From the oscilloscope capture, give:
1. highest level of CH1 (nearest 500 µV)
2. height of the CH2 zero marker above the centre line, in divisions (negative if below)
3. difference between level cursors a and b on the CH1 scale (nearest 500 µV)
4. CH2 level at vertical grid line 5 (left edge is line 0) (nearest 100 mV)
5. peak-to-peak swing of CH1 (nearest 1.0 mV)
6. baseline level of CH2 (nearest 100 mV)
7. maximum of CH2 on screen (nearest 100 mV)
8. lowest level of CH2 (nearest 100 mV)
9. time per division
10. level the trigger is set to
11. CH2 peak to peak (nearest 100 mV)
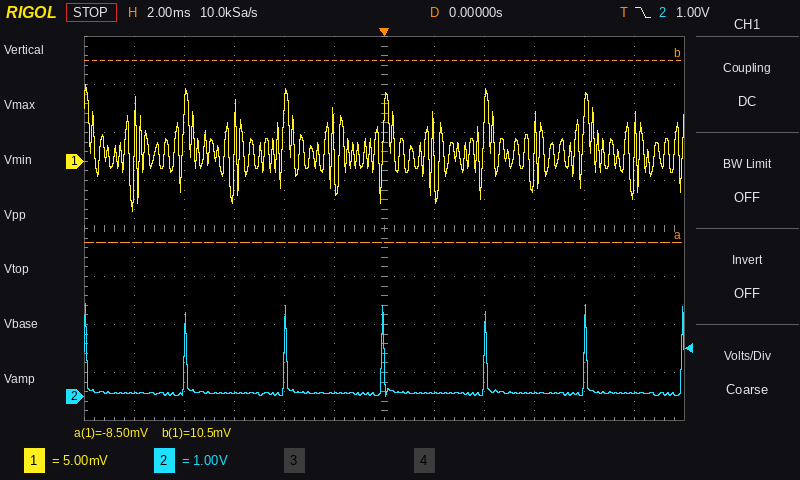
8.0 mV
-3.5 div
19.0 mV
100 mV
13.0 mV
100 mV
1.9 V
0.0 V
2 ms
1.00 V
1.9 V
